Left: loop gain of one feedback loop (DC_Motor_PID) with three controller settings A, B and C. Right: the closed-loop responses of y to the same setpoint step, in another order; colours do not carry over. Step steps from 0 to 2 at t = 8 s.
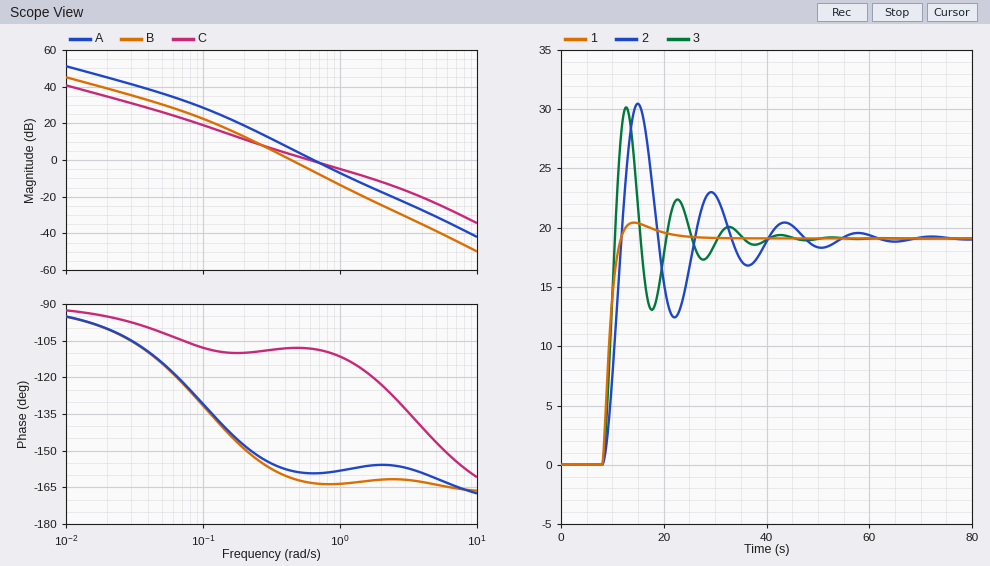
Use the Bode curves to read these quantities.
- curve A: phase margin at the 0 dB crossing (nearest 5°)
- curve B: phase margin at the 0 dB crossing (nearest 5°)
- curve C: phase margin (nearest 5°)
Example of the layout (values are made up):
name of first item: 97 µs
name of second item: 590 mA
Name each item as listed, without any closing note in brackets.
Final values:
curve A: phase margin at the 0 dB crossing: 20°
curve B: phase margin at the 0 dB crossing: 20°
curve C: phase margin: 70°
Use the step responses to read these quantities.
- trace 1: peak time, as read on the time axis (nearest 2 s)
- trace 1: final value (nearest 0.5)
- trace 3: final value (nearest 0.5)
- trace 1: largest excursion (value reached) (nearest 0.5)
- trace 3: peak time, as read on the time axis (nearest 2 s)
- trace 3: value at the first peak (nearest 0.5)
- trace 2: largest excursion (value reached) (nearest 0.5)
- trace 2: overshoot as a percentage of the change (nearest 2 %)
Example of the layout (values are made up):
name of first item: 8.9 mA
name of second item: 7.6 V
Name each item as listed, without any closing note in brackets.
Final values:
trace 1: peak time, as read on the time axis: 14 s
trace 1: final value: 19.0
trace 3: final value: 19.0
trace 1: largest excursion (value reached): 20.5
trace 3: peak time, as read on the time axis: 12 s
trace 3: value at the first peak: 30.0
trace 2: largest excursion (value reached): 30.5
trace 2: overshoot as a percentage of the change: 60 %
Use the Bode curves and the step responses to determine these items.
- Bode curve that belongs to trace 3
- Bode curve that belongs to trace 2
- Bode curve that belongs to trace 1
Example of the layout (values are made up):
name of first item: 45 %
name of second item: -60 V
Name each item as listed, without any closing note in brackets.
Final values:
Bode curve that belongs to trace 3: A
Bode curve that belongs to trace 2: B
Bode curve that belongs to trace 1: C
